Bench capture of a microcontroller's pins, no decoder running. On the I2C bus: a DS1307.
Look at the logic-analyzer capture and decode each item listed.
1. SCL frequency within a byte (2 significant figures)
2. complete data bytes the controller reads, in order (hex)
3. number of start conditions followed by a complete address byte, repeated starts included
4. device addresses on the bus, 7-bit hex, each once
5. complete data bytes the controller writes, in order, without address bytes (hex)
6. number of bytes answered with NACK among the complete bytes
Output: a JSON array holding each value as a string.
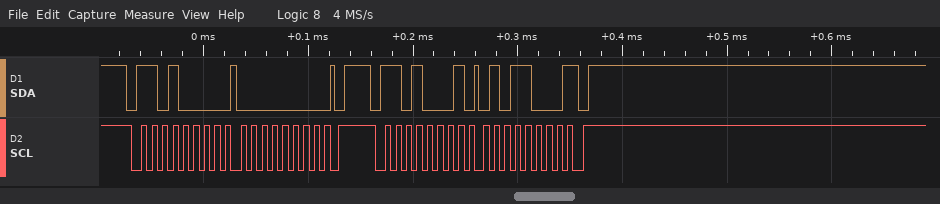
["100 kHz", "58", "2", "0x68", "00", "1"]
